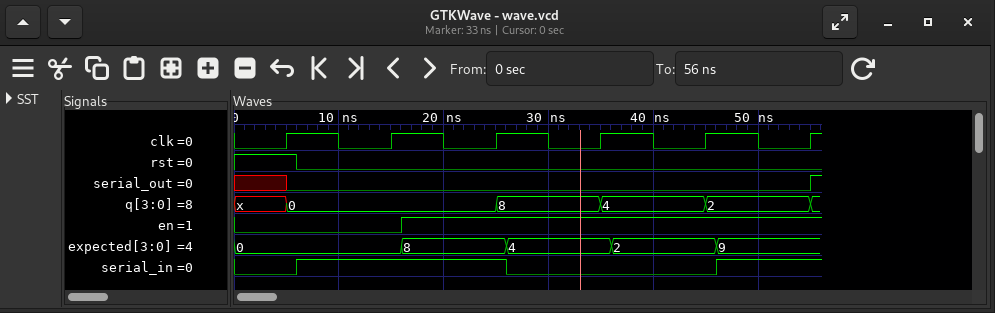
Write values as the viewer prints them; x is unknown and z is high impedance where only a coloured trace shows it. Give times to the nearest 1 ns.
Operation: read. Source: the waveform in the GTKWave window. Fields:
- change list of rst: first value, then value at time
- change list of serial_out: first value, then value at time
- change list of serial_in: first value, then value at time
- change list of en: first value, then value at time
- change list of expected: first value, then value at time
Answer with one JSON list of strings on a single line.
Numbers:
["1, 0 at 6 ns", "x, 0 at 5 ns, 1 at 55 ns", "0, 1 at 6 ns, 0 at 26 ns, 1 at 46 ns", "0, 1 at 16 ns", "0, 8 at 16 ns, 4 at 26 ns, 2 at 36 ns, 9 at 46 ns"]
